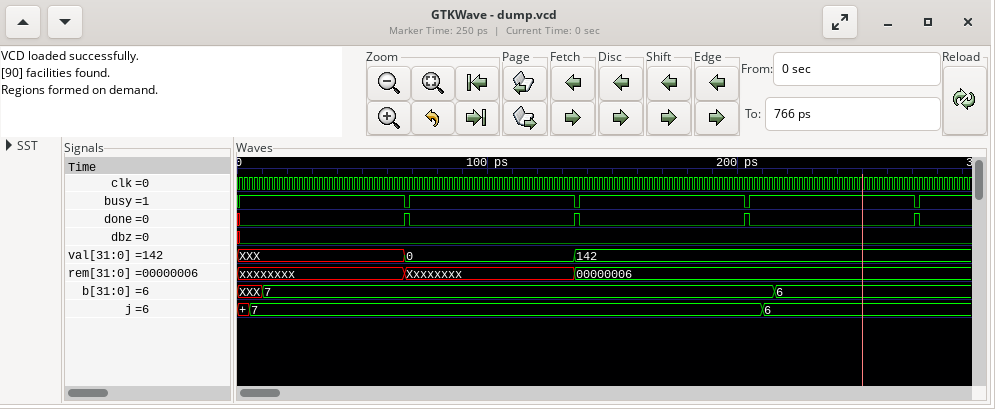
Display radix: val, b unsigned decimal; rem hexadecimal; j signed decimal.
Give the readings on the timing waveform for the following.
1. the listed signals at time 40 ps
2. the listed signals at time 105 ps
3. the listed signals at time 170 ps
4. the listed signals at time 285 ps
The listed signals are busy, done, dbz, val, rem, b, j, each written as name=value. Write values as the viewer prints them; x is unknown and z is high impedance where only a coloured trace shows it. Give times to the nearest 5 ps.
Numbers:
busy=1, done=0, dbz=0, val=XXX, rem=xxxxxxxx, b=7, j=7
busy=1, done=0, dbz=0, val=0, rem=Xxxxxxxx, b=7, j=7
busy=1, done=0, dbz=0, val=142, rem=00000006, b=7, j=7
busy=1, done=0, dbz=0, val=142, rem=00000006, b=6, j=6
